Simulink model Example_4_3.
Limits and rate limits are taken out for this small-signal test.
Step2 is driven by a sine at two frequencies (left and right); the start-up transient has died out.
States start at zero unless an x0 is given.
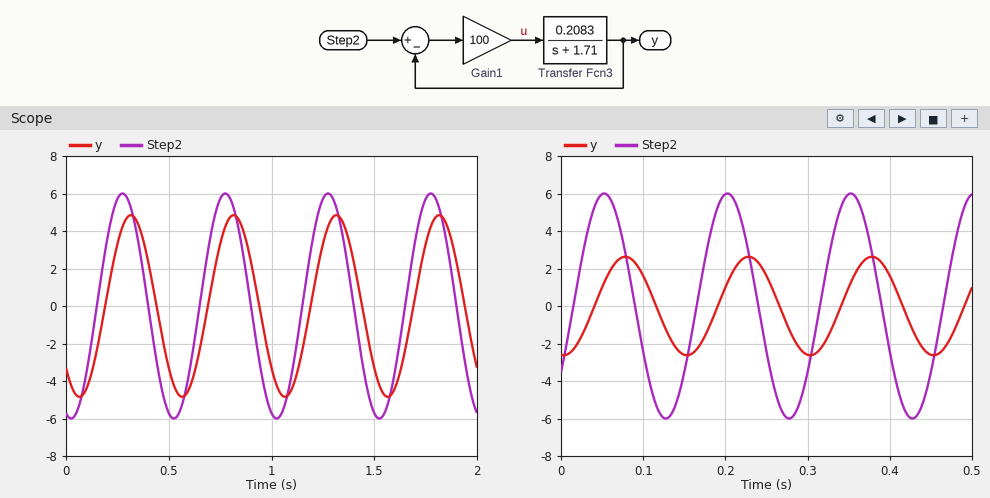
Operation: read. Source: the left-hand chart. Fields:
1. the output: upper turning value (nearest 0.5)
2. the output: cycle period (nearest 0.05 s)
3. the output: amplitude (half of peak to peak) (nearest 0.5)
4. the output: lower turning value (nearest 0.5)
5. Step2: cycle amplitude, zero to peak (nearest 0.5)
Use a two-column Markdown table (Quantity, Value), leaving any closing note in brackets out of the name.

| Quantity | Value |
|---|---|
| the output: upper turning value | 5.0 |
| the output: cycle period | 0.50 s |
| the output: amplitude (half of peak to peak) | 5.0 |
| the output: lower turning value | -5.0 |
| Step2: cycle amplitude, zero to peak | 6.0 |
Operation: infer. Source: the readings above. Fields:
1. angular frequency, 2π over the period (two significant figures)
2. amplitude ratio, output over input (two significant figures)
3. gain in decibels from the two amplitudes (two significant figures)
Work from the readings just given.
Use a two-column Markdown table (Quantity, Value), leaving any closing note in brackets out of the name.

| Quantity | Value |
|---|---|
| angular frequency, 2π over the period | 13 rad/s |
| amplitude ratio, output over input | 0.83 |
| gain in decibels from the two amplitudes | -1.6 dB |
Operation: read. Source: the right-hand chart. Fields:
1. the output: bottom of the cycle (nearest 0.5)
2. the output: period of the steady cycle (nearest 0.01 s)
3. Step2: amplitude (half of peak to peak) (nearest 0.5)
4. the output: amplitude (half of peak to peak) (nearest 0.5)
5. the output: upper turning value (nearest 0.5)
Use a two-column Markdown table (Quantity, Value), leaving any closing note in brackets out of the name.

| Quantity | Value |
|---|---|
| the output: bottom of the cycle | -2.5 |
| the output: period of the steady cycle | 0.15 s |
| Step2: amplitude (half of peak to peak) | 6.0 |
| the output: amplitude (half of peak to peak) | 2.5 |
| the output: upper turning value | 2.5 |
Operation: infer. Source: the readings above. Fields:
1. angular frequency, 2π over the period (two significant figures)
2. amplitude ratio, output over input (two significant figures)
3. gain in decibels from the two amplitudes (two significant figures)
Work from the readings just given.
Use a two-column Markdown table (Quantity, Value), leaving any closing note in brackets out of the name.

| Quantity | Value |
|---|---|
| angular frequency, 2π over the period | 42 rad/s |
| amplitude ratio, output over input | 0.42 |
| gain in decibels from the two amplitudes | -7.6 dB |
